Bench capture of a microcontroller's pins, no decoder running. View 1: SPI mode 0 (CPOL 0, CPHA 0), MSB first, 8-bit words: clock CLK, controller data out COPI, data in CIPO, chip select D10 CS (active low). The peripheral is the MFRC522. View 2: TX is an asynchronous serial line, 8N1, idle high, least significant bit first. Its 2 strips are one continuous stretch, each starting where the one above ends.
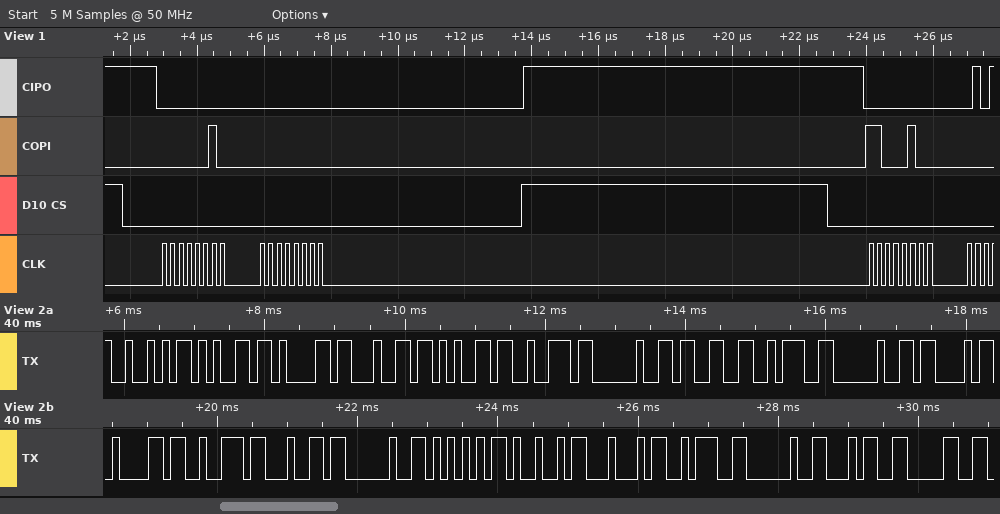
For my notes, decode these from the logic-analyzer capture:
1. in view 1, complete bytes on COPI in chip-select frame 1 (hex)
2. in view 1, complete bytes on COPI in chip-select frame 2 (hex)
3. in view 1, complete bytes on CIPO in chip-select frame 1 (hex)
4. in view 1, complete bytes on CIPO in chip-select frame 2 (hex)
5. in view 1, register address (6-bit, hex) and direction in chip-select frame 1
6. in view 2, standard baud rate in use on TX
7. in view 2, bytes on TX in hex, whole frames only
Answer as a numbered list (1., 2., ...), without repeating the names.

1. 0x02 0x00
2. 0xC4
3. 0x00 0x00
4. 0x00
5. 0x01 write
6. 9600 baud
7. 52 65 61 64 65 72 20 33 3A 20 43 61 72 64 20 55 49 44 3A 20 34 30
